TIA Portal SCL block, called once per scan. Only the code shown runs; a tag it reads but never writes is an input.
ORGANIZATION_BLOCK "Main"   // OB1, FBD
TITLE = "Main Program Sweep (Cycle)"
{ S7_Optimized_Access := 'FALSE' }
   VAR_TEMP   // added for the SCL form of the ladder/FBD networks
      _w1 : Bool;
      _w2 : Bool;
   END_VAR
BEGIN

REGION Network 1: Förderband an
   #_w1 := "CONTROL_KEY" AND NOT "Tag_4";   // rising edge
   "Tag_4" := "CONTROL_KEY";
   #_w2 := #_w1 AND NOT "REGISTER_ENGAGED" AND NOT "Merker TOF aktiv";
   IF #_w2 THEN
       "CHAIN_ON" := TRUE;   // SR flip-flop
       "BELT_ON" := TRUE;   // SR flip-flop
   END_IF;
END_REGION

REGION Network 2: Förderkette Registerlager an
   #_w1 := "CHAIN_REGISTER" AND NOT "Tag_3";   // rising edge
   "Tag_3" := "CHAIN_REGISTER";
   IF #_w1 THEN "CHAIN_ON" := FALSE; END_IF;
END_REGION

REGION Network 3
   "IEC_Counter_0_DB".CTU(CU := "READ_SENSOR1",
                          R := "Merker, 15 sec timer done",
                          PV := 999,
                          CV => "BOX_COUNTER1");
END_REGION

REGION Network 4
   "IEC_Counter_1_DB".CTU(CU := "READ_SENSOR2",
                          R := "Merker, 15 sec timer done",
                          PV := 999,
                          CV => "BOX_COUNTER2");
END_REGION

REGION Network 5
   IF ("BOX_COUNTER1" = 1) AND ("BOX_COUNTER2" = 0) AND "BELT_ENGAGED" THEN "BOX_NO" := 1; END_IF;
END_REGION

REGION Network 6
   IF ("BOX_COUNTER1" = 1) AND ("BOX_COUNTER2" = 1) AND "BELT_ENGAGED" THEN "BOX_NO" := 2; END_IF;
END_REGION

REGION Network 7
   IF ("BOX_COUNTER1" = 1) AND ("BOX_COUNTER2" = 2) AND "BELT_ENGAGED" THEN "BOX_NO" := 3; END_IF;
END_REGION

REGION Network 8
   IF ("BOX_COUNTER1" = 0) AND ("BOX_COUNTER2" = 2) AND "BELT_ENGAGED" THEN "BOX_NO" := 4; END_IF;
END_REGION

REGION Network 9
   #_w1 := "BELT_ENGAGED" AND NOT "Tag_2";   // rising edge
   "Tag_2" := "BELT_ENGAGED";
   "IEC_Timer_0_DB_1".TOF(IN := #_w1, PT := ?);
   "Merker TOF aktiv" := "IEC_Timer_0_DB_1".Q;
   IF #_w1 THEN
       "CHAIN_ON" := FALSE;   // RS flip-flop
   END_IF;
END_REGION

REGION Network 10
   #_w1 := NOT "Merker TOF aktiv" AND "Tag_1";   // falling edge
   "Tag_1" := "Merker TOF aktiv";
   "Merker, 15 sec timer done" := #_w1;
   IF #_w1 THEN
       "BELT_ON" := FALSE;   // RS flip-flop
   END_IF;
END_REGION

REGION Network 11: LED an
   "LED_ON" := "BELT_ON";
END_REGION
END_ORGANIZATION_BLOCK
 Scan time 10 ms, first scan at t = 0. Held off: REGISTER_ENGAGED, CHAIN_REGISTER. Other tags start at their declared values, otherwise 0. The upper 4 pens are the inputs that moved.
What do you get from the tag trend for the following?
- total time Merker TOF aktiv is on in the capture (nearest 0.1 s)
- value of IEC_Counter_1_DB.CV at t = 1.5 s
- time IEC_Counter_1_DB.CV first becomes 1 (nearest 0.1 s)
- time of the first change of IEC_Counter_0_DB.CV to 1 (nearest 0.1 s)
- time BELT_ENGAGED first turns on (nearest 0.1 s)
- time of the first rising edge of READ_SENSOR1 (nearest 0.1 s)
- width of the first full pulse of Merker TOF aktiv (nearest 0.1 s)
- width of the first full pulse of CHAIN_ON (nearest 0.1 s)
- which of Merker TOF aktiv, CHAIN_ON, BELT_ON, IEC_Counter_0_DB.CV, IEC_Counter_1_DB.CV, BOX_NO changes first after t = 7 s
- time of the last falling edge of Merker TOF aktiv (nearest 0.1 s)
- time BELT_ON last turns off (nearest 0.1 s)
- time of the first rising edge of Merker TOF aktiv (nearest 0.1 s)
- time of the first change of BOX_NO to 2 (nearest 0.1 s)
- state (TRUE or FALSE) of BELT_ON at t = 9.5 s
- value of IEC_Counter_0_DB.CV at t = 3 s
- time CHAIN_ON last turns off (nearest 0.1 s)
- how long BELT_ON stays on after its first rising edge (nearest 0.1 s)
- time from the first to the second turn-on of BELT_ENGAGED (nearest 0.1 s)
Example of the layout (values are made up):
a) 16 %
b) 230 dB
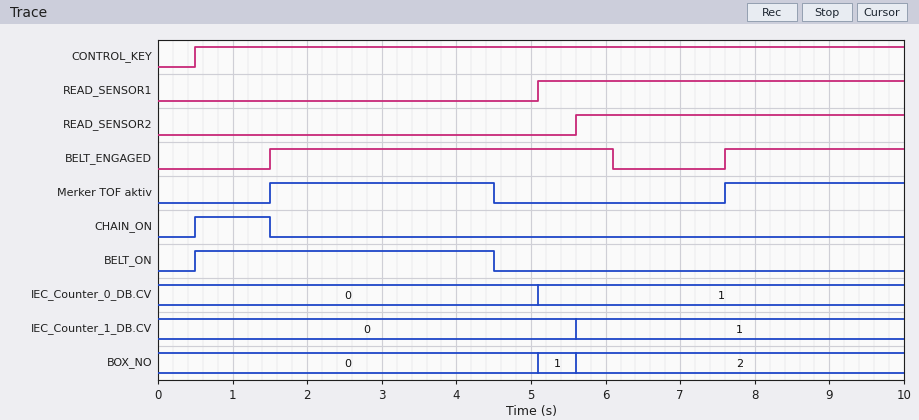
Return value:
a) 5.4 s
b) 0
c) 5.6 s
d) 5.1 s
e) 1.5 s
f) 5.1 s
g) 3.0 s
h) 1.0 s
i) Merker TOF aktiv
j) 4.5 s
k) 4.5 s
l) 1.5 s
m) 5.6 s
n) FALSE
o) 0
p) 1.5 s
q) 4.0 s
r) 6.1 s
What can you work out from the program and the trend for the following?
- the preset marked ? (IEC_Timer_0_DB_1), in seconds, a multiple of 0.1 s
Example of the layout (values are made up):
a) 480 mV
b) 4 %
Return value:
a) 3.0 s
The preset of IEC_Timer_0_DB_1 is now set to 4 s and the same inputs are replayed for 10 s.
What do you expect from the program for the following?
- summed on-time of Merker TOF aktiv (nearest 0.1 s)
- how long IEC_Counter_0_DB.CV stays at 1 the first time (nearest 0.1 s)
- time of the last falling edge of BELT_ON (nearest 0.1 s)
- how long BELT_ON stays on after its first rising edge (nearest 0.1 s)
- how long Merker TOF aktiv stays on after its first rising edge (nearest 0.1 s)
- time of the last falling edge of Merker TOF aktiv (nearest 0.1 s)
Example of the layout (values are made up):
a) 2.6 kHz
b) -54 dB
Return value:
a) 6.4 s
b) 0.4 s
c) 5.5 s
d) 5.0 s
e) 4.0 s
f) 5.5 s
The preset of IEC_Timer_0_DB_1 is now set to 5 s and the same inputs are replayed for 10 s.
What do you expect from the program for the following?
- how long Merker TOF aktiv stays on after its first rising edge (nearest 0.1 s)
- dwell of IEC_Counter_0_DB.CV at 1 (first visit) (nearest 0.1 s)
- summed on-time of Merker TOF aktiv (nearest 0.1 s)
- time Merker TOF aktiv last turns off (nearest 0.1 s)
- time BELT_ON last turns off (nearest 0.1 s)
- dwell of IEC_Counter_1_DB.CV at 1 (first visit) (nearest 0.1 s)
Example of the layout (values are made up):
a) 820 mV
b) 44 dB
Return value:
a) 5.0 s
b) 1.4 s
c) 7.4 s
d) 6.5 s
e) 6.5 s
f) 0.9 s
